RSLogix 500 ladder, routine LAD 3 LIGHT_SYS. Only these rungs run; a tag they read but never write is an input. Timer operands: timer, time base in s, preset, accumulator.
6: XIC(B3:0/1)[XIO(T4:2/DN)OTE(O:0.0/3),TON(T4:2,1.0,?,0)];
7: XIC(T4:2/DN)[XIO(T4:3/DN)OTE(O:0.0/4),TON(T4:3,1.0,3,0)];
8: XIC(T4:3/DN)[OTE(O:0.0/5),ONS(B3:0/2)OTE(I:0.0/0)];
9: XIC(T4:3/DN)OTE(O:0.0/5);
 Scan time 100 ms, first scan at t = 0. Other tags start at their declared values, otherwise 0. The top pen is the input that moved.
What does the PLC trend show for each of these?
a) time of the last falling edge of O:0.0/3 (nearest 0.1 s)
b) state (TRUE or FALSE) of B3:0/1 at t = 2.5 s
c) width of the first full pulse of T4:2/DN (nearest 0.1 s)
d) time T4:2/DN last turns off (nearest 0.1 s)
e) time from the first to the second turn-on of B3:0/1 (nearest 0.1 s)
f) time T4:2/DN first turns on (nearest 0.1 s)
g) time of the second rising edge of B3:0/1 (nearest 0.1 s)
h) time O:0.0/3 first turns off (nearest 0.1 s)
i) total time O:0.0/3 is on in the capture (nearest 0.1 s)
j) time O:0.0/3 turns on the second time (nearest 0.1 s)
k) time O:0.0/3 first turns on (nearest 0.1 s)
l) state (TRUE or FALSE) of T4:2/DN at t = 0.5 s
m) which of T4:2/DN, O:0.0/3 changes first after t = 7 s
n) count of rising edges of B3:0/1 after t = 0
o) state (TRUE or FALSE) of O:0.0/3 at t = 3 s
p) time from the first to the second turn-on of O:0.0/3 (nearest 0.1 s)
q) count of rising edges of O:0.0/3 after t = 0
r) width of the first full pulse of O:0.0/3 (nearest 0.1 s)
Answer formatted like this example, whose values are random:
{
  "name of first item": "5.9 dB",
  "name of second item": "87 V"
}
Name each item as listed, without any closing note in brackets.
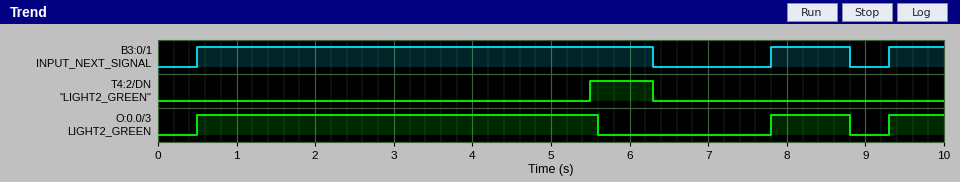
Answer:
{
  "time of the last falling edge of O:0.0/3": "8.8 s",
  "state (TRUE or FALSE) of B3:0/1 at t = 2.5 s": "TRUE",
  "width of the first full pulse of T4:2/DN": "0.8 s",
  "time T4:2/DN last turns off": "6.3 s",
  "time from the first to the second turn-on of B3:0/1": "7.3 s",
  "time T4:2/DN first turns on": "5.5 s",
  "time of the second rising edge of B3:0/1": "7.8 s",
  "time O:0.0/3 first turns off": "5.6 s",
  "total time O:0.0/3 is on in the capture": "6.8 s",
  "time O:0.0/3 turns on the second time": "7.8 s",
  "time O:0.0/3 first turns on": "0.5 s",
  "state (TRUE or FALSE) of T4:2/DN at t = 0.5 s": "FALSE",
  "which of T4:2/DN, O:0.0/3 changes first after t = 7 s": "O:0.0/3",
  "count of rising edges of B3:0/1 after t = 0": "3",
  "state (TRUE or FALSE) of O:0.0/3 at t = 3 s": "TRUE",
  "time from the first to the second turn-on of O:0.0/3": "7.3 s",
  "count of rising edges of O:0.0/3 after t = 0": "3",
  "width of the first full pulse of O:0.0/3": "5.1 s"
}
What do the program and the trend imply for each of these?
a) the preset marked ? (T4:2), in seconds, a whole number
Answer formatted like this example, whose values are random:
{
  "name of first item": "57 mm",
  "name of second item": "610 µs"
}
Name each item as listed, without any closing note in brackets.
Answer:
{
  "the preset marked ? (T4:2), in seconds, a whole number": "5 s"
}
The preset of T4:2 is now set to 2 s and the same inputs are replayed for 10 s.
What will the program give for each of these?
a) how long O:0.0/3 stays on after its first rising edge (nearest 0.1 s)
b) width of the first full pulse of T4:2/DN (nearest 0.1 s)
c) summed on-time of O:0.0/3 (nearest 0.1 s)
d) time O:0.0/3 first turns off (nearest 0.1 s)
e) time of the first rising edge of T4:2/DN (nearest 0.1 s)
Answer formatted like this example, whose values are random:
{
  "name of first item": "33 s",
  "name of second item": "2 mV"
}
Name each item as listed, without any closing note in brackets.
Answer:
{
  "how long O:0.0/3 stays on after its first rising edge": "2.1 s",
  "width of the first full pulse of T4:2/DN": "3.8 s",
  "summed on-time of O:0.0/3": "3.8 s",
  "time O:0.0/3 first turns off": "2.6 s",
  "time of the first rising edge of T4:2/DN": "2.5 s"
}
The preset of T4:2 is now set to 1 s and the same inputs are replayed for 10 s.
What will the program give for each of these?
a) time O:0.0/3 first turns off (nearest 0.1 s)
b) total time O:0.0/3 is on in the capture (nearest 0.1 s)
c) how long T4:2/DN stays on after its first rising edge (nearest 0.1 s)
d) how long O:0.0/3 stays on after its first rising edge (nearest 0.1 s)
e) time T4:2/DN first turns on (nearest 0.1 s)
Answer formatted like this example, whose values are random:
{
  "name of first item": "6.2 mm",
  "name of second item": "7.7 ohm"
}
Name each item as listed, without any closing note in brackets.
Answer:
{
  "time O:0.0/3 first turns off": "1.6 s",
  "total time O:0.0/3 is on in the capture": "2.8 s",
  "how long T4:2/DN stays on after its first rising edge": "4.8 s",
  "how long O:0.0/3 stays on after its first rising edge": "1.1 s",
  "time T4:2/DN first turns on": "1.5 s"
}
